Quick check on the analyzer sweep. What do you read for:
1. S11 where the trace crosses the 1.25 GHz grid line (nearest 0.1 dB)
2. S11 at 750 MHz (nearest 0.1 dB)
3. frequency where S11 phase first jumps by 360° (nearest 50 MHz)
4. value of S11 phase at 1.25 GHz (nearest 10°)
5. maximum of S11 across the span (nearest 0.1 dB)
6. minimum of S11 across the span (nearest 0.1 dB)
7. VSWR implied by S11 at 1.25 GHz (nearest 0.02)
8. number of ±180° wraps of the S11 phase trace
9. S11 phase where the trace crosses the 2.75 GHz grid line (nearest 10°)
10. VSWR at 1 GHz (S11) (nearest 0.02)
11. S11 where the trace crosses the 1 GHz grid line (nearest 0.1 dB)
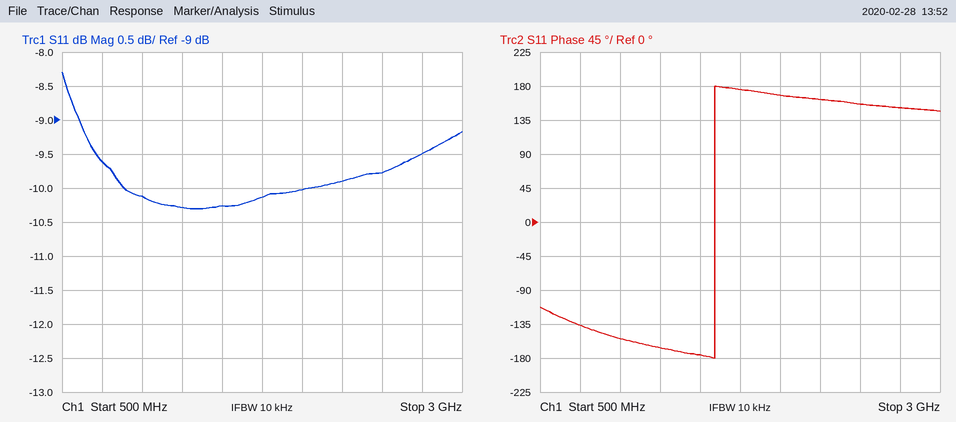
-10.3 dB
-9.6 dB
1.60 GHz
-170°
-8.3 dB
-10.3 dB
1.88
1
150°
1.90
-10.1 dB
